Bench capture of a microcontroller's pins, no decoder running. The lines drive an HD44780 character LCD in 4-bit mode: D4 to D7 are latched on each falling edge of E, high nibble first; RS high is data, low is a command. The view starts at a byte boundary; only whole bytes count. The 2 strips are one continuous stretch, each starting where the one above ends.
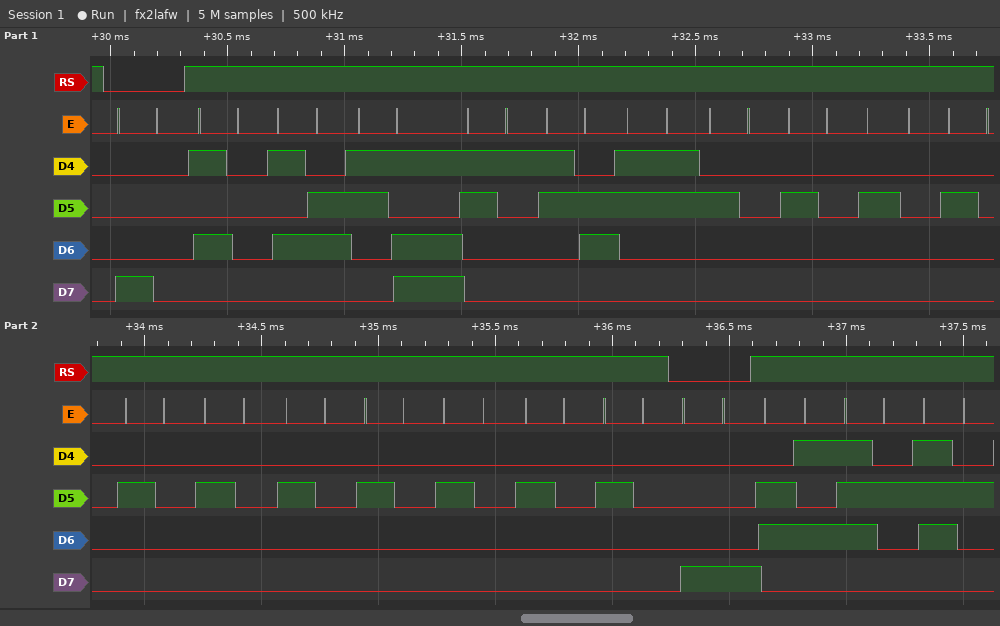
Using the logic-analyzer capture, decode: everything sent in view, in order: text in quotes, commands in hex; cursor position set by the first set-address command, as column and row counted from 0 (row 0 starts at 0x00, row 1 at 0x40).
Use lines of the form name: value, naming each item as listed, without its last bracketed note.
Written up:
everything sent in view, in order: text in quotes, commands in hex: 0x80 "PV=163           " 0x88 "err"
cursor position set by the first set-address command, as column and row counted from 0: column 0, row 0
